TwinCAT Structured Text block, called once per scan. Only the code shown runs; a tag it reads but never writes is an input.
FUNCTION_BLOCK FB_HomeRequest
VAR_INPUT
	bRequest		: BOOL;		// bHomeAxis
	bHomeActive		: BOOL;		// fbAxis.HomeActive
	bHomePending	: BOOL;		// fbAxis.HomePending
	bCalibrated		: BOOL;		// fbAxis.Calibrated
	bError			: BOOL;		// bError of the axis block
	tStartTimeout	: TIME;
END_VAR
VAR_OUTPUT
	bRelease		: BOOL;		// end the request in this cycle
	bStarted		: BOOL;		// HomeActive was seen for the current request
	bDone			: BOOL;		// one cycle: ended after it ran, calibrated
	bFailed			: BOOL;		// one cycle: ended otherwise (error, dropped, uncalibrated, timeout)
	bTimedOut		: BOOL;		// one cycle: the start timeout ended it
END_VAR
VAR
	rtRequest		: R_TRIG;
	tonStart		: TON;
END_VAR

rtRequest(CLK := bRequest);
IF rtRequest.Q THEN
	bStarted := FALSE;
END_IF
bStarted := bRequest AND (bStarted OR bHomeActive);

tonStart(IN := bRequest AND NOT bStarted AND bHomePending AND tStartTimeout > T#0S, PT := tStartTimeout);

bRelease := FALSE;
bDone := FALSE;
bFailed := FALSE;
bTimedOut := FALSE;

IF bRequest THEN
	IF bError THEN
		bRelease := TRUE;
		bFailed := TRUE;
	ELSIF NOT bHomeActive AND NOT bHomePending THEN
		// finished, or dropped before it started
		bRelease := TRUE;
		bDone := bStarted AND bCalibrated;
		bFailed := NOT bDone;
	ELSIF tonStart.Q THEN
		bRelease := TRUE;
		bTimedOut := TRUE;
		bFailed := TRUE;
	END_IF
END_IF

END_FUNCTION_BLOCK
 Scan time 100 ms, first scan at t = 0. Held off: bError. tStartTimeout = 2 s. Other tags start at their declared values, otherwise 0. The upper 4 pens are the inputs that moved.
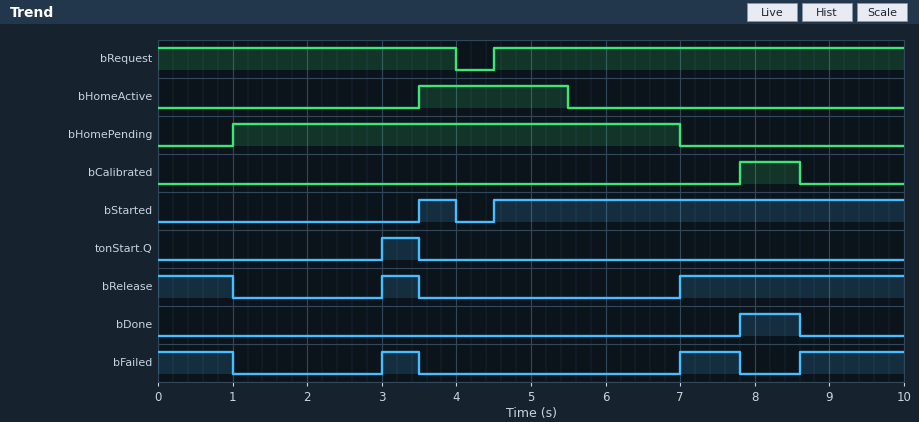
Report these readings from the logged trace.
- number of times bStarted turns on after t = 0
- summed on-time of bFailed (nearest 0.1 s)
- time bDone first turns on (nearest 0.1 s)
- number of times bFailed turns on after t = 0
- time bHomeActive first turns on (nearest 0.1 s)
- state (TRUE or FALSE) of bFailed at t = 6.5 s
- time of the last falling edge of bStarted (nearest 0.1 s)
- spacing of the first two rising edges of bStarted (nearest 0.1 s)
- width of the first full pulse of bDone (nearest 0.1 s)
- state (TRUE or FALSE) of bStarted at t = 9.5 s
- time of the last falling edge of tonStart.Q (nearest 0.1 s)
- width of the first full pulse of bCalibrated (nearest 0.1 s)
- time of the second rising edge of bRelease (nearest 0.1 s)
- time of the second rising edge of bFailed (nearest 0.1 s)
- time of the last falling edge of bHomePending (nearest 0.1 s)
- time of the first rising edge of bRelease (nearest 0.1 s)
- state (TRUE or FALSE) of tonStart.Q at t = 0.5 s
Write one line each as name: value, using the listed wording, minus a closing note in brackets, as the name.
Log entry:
number of times bStarted turns on after t = 0: 2
summed on-time of bFailed: 3.7 s
time bDone first turns on: 7.8 s
number of times bFailed turns on after t = 0: 3
time bHomeActive first turns on: 3.5 s
state (TRUE or FALSE) of bFailed at t = 6.5 s: FALSE
time of the last falling edge of bStarted: 4.0 s
spacing of the first two rising edges of bStarted: 1.0 s
width of the first full pulse of bDone: 0.8 s
state (TRUE or FALSE) of bStarted at t = 9.5 s: TRUE
time of the last falling edge of tonStart.Q: 3.5 s
width of the first full pulse of bCalibrated: 0.8 s
time of the second rising edge of bRelease: 7.0 s
time of the second rising edge of bFailed: 7.0 s
time of the last falling edge of bHomePending: 7.0 s
time of the first rising edge of bRelease: 3.0 s
state (TRUE or FALSE) of tonStart.Q at t = 0.5 s: FALSE
